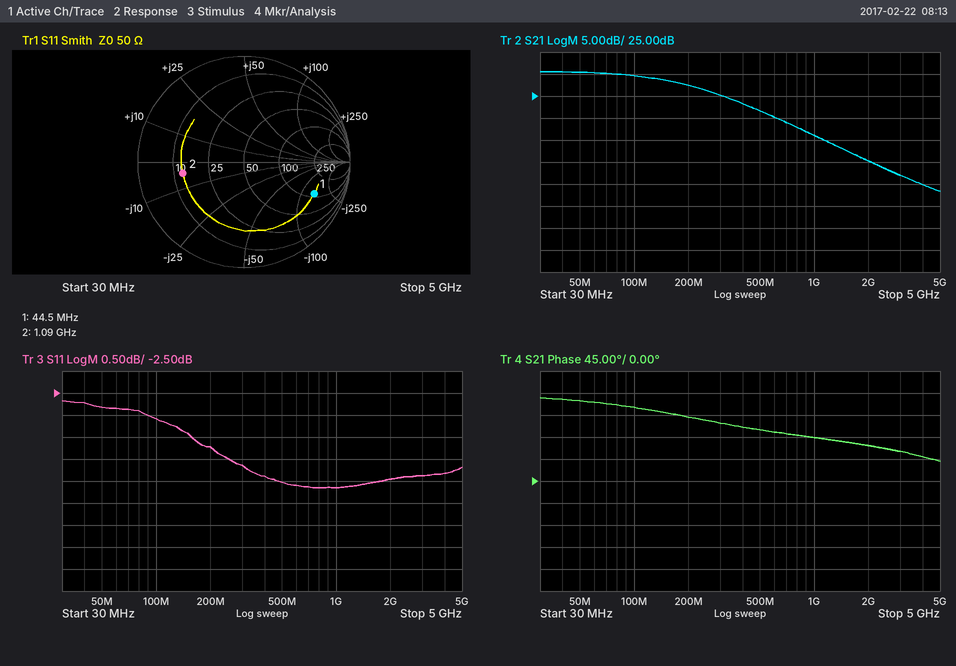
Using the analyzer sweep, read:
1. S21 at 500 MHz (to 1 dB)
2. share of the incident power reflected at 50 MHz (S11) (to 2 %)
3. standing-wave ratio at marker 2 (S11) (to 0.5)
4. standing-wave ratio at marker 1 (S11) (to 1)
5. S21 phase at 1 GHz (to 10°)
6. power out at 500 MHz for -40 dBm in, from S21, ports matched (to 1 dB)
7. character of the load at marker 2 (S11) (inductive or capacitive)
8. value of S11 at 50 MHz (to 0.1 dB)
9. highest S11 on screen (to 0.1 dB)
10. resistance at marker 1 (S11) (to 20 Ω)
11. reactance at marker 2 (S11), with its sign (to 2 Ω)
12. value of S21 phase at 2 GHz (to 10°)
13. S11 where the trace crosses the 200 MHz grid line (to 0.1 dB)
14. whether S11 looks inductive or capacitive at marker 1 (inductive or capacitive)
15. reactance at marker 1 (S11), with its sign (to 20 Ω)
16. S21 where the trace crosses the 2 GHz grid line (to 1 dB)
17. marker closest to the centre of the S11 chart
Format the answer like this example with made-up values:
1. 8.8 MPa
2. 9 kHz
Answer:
1. 22 dB
2. 52 %
3. 4.0
4. 6
5. 90°
6. -18 dBm
7. capacitive
8. -2.8 dB
9. -2.7 dB
10. 120 Ω
11. -4 Ω
12. 70°
13. -3.7 dB
14. capacitive
15. -140 Ω
16. 10 dB
17. marker 2
